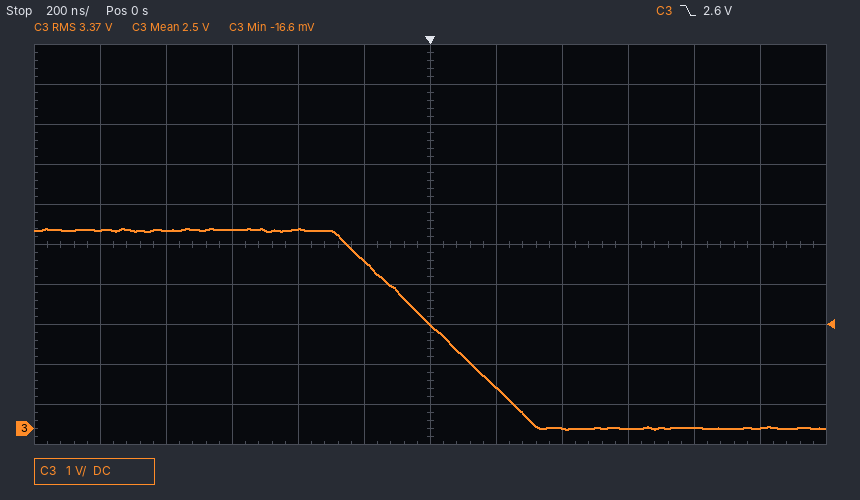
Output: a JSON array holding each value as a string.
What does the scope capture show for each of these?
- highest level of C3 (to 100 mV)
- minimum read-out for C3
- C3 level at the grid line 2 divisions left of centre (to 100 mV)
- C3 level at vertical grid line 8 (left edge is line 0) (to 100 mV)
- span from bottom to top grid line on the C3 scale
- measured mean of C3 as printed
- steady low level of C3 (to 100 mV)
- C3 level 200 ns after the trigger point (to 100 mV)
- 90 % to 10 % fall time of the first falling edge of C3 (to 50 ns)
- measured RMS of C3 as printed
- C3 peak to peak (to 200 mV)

["5.0 V", "-16.6 mV", "5.0 V", "0.0 V", "10 V", "2.5 V", "0.0 V", "1.0 V", "500 ns", "3.37 V", "5.0 V"]
